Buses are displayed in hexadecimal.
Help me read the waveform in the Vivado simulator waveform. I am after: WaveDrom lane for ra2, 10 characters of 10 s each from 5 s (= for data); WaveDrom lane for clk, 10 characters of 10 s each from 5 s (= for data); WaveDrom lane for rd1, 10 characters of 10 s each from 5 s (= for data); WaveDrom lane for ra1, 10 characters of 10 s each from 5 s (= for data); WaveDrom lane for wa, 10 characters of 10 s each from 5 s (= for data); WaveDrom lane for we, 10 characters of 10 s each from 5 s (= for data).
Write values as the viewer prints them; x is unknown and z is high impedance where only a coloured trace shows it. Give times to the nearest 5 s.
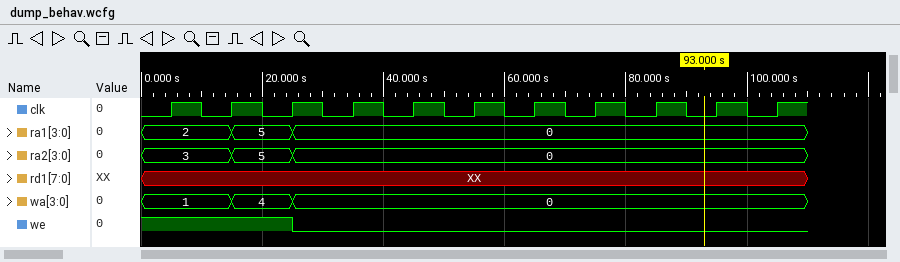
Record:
{name: 'ra2', wave: '===.......', data: '3 5 0'}
{name: 'clk', wave: 'p.........'}
{name: 'rd1', wave: 'x.........'}
{name: 'ra1', wave: '===.......', data: '2 5 0'}
{name: 'wa', wave: '===.......', data: '1 4 0'}
{name: 'we', wave: '1.0.......'}
